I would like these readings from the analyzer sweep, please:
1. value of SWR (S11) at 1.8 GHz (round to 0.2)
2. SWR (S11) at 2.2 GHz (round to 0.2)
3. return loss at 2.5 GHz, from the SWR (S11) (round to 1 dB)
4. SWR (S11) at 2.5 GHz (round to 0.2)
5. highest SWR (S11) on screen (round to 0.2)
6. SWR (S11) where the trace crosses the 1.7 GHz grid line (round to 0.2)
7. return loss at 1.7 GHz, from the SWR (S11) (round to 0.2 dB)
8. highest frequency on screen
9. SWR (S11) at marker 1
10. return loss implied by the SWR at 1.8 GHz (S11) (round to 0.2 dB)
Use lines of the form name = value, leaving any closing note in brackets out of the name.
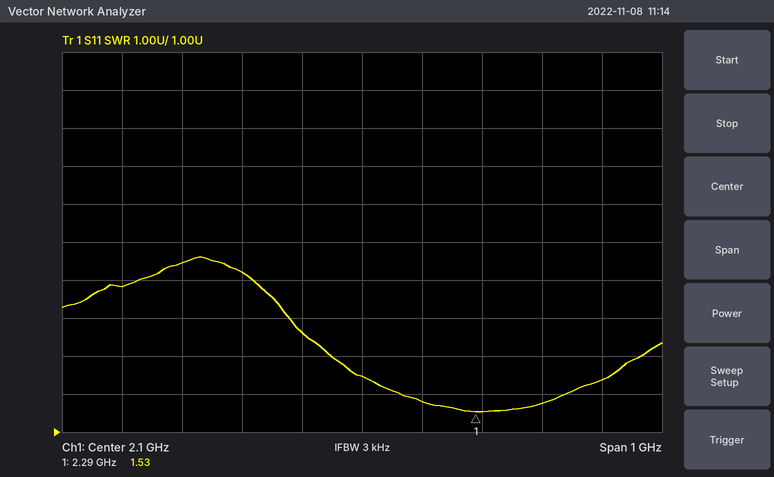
value of SWR (S11) at 1.8 GHz = 5.4
SWR (S11) at 2.2 GHz = 1.8
return loss at 2.5 GHz, from the SWR (S11) = 8 dB
SWR (S11) at 2.5 GHz = 2.4
highest SWR (S11) on screen = 5.6
SWR (S11) where the trace crosses the 1.7 GHz grid line = 4.8
return loss at 1.7 GHz, from the SWR (S11) = 3.6 dB
highest frequency on screen = 2.6 GHz
SWR (S11) at marker 1 = 1.53
return loss implied by the SWR at 1.8 GHz (S11) = 3.2 dB
